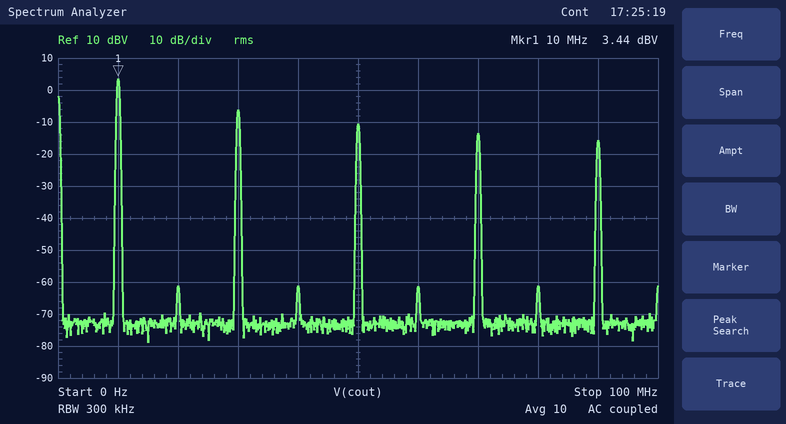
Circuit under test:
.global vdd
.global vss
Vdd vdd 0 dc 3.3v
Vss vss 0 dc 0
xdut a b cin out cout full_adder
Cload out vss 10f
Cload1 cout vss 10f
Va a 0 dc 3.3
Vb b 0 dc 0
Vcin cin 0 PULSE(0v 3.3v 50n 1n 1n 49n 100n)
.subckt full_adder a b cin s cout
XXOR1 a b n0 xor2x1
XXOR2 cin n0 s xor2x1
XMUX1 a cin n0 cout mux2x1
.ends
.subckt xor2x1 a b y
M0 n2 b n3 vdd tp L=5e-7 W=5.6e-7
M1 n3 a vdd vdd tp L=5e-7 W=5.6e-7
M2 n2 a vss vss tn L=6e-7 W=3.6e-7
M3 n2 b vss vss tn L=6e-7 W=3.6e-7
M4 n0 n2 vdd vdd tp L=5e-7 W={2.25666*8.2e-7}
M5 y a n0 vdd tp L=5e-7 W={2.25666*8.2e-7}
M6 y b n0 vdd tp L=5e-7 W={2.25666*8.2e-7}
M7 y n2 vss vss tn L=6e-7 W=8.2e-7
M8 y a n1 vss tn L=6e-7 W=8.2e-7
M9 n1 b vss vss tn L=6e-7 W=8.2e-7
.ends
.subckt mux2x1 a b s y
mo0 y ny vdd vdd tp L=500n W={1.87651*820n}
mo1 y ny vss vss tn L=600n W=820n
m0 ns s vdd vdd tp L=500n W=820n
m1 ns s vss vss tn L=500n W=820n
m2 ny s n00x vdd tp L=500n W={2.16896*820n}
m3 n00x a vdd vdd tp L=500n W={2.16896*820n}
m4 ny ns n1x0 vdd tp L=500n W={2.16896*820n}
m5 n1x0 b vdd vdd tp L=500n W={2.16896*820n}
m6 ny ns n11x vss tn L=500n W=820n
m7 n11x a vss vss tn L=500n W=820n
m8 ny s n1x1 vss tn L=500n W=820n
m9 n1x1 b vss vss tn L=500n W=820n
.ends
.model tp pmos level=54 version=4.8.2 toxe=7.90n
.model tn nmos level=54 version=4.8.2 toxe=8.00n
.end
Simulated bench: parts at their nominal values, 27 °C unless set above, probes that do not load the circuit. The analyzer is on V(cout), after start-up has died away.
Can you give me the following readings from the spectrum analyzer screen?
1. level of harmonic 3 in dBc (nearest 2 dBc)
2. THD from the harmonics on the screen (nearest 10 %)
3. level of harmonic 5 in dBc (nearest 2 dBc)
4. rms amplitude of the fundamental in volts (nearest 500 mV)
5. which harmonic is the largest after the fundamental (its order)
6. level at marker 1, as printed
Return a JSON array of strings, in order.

["-10 dBc", "40 %", "-14 dBc", "1.5 V", "3", "3.44 dBV"]
